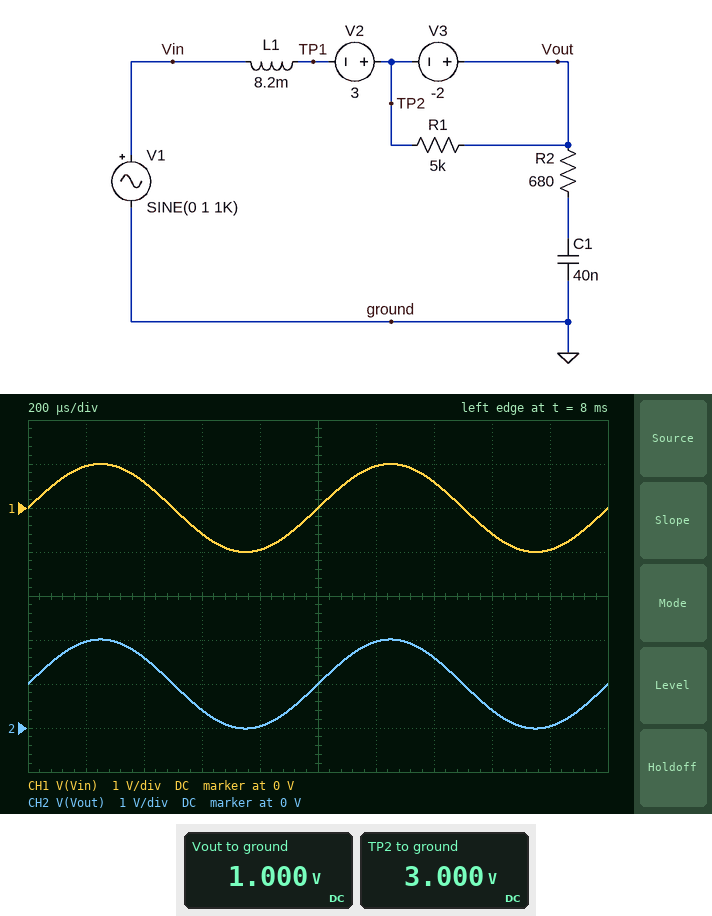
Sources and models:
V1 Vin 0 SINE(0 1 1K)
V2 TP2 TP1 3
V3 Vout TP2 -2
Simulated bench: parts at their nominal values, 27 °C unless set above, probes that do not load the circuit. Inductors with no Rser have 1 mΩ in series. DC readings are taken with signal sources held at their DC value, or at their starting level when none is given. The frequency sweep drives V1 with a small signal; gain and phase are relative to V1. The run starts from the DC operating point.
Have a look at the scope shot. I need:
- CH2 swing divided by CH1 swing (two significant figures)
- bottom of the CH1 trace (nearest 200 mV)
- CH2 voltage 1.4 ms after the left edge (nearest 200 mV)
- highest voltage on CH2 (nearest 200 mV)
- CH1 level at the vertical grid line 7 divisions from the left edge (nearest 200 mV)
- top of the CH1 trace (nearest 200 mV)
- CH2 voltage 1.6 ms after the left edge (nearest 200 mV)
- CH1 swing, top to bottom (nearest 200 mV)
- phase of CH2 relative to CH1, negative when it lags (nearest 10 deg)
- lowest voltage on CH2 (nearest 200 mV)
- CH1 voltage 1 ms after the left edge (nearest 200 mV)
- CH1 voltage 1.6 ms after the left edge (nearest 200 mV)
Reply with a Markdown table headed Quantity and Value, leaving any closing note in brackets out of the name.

| Quantity | Value |
|---|---|
| CH2 swing divided by CH1 swing | 1.0 |
| bottom of the CH1 trace | -1.0 V |
| CH2 voltage 1.4 ms after the left edge | 1.6 V |
| highest voltage on CH2 | 2.0 V |
| CH1 level at the vertical grid line 7 divisions from the left edge | 600 mV |
| top of the CH1 trace | 1.0 V |
| CH2 voltage 1.6 ms after the left edge | 400 mV |
| CH1 swing, top to bottom | 2.0 V |
| phase of CH2 relative to CH1, negative when it lags | 0 deg |
| lowest voltage on CH2 | 0 V |
| CH1 voltage 1 ms after the left edge | 0 V |
| CH1 voltage 1.6 ms after the left edge | -600 mV |
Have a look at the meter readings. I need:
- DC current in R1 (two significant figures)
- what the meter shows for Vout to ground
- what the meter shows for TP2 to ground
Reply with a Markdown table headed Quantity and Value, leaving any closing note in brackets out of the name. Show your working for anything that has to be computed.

| Quantity | Value |
|---|---|
| DC current in R1 | (3 V - 1 V) / 5 kΩ = 400 µA |
| what the meter shows for Vout to ground | 1.000 V |
| what the meter shows for TP2 to ground | 3.000 V |
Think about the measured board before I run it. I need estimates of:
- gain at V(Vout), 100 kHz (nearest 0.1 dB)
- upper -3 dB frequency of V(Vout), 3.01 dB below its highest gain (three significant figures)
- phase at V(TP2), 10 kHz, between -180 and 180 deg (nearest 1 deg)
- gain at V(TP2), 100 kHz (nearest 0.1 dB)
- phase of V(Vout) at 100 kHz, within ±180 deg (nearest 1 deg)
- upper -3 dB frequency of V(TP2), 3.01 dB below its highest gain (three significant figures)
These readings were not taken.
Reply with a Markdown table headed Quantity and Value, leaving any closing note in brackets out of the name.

| Quantity | Value |
|---|---|
| gain at V(Vout), 100 kHz | -17.6 dB |
| upper -3 dB frequency of V(Vout), 3.01 dB below its highest gain | 14.6 kHz |
| phase at V(TP2), 10 kHz, between -180 and 180 deg | -40 deg |
| gain at V(TP2), 100 kHz | -17.6 dB |
| phase of V(Vout) at 100 kHz, within ±180 deg | -86 deg |
| upper -3 dB frequency of V(TP2), 3.01 dB below its highest gain | 14.6 kHz |
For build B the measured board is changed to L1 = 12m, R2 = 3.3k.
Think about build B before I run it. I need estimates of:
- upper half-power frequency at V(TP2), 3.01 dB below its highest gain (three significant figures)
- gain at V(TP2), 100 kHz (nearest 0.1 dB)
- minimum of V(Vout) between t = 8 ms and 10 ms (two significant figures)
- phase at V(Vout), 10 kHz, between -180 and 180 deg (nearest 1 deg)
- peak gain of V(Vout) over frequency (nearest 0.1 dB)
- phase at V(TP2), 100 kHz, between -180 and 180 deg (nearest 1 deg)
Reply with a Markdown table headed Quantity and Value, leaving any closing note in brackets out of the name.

| Quantity | Value |
|---|---|
| upper half-power frequency at V(TP2), 3.01 dB below its highest gain | 43.1 kHz |
| gain at V(TP2), 100 kHz | -7.9 dB |
| minimum of V(Vout) between t = 8 ms and 10 ms | -11 mV |
| phase at V(Vout), 10 kHz, between -180 and 180 deg | -13 deg |
| peak gain of V(Vout) over frequency | 0.2 dB |
| phase at V(TP2), 100 kHz, between -180 and 180 deg | -67 deg |
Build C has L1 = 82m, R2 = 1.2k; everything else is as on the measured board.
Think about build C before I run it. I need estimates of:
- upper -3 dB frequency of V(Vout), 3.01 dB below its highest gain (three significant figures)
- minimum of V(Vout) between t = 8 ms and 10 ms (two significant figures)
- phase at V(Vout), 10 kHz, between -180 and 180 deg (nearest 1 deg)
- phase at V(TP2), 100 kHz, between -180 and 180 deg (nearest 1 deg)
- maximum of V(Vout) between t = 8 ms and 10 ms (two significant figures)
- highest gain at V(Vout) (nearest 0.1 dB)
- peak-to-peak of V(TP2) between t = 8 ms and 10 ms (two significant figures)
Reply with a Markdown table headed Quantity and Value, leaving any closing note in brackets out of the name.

| Quantity | Value |
|---|---|
| upper -3 dB frequency of V(Vout), 3.01 dB below its highest gain | 3.63 kHz |
| minimum of V(Vout) between t = 8 ms and 10 ms | -130 mV |
| phase at V(Vout), 10 kHz, between -180 and 180 deg | -94 deg |
| phase at V(TP2), 100 kHz, between -180 and 180 deg | -91 deg |
| maximum of V(Vout) between t = 8 ms and 10 ms | 2.1 V |
| highest gain at V(Vout) | 4.1 dB |
| peak-to-peak of V(TP2) between t = 8 ms and 10 ms | 2.3 V |
